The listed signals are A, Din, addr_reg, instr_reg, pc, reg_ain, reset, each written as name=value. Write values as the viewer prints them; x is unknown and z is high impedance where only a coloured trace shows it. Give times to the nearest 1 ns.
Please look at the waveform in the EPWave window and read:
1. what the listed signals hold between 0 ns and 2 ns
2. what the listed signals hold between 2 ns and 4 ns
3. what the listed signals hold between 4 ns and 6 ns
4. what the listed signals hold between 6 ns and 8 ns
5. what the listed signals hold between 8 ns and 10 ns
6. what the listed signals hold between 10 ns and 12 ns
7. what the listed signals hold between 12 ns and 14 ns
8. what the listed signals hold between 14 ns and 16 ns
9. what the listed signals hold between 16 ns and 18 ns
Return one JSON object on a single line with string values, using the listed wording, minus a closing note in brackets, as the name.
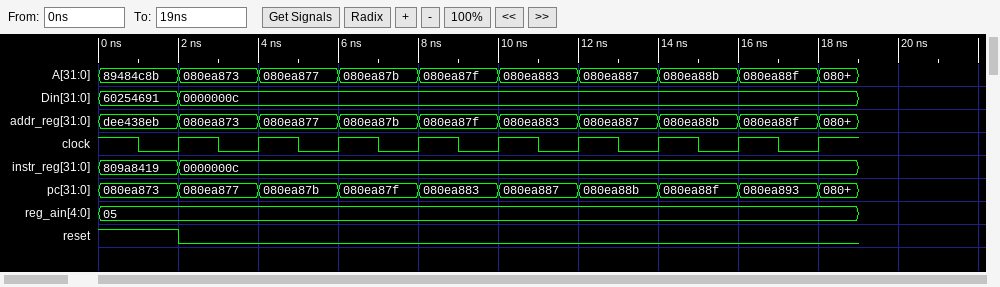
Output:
{"what the listed signals hold between 0 ns and 2 ns": "A=89484c8b, Din=60254691, addr_reg=dee438eb, instr_reg=809a8419, pc=080ea873, reg_ain=05, reset=1", "what the listed signals hold between 2 ns and 4 ns": "A=080ea873, Din=0000000c, addr_reg=080ea873, instr_reg=0000000c, pc=080ea877, reg_ain=05, reset=0", "what the listed signals hold between 4 ns and 6 ns": "A=080ea877, Din=0000000c, addr_reg=080ea877, instr_reg=0000000c, pc=080ea87b, reg_ain=05, reset=0", "what the listed signals hold between 6 ns and 8 ns": "A=080ea87b, Din=0000000c, addr_reg=080ea87b, instr_reg=0000000c, pc=080ea87f, reg_ain=05, reset=0", "what the listed signals hold between 8 ns and 10 ns": "A=080ea87f, Din=0000000c, addr_reg=080ea87f, instr_reg=0000000c, pc=080ea883, reg_ain=05, reset=0", "what the listed signals hold between 10 ns and 12 ns": "A=080ea883, Din=0000000c, addr_reg=080ea883, instr_reg=0000000c, pc=080ea887, reg_ain=05, reset=0", "what the listed signals hold between 12 ns and 14 ns": "A=080ea887, Din=0000000c, addr_reg=080ea887, instr_reg=0000000c, pc=080ea88b, reg_ain=05, reset=0", "what the listed signals hold between 14 ns and 16 ns": "A=080ea88b, Din=0000000c, addr_reg=080ea88b, instr_reg=0000000c, pc=080ea88f, reg_ain=05, reset=0", "what the listed signals hold between 16 ns and 18 ns": "A=080ea88f, Din=0000000c, addr_reg=080ea88f, instr_reg=0000000c, pc=080ea893, reg_ain=05, reset=0"}
